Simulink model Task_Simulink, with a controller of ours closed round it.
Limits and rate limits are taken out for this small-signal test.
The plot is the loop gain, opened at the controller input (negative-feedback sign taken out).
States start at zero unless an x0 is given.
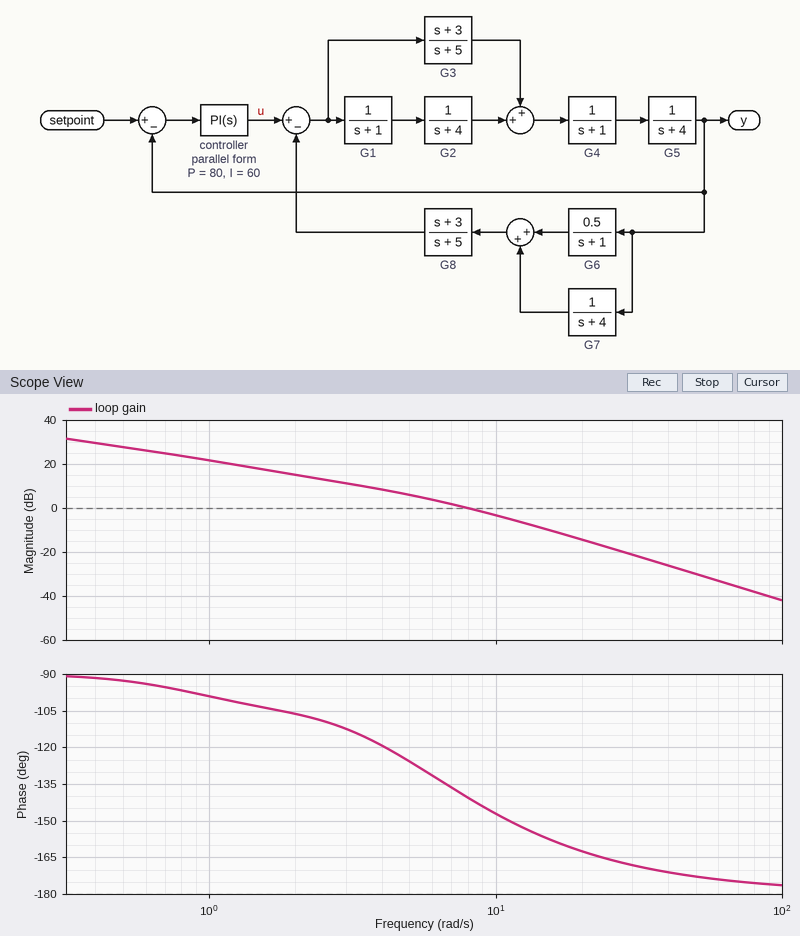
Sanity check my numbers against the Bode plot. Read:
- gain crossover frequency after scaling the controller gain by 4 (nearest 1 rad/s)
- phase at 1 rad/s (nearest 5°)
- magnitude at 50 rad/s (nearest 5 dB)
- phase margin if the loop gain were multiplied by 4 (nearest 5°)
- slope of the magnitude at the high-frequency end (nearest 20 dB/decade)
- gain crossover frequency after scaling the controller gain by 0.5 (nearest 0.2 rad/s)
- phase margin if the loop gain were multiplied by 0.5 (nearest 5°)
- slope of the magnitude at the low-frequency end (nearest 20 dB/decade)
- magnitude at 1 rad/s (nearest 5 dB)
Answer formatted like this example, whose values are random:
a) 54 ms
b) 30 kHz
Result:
a) 17 rad/s
b) -100°
c) -30 dB
d) 20°
e) -40 dB/decade
f) 5.0 rad/s
g) 55°
h) -20 dB/decade
i) 20 dB
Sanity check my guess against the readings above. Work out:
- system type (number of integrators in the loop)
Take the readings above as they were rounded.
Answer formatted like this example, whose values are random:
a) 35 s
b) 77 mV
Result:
a) 1
